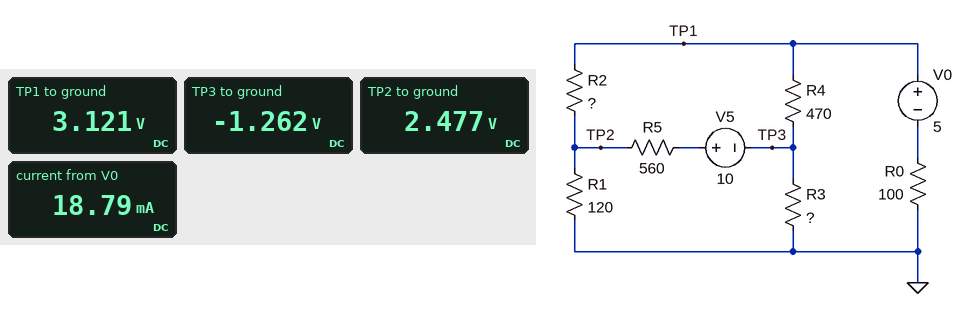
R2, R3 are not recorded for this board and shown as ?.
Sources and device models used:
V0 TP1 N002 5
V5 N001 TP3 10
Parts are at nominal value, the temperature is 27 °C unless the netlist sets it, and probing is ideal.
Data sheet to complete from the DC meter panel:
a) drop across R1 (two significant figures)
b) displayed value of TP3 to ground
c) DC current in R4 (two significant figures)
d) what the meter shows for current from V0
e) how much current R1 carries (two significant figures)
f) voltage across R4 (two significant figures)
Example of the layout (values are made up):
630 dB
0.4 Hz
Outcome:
2.5 V
-1.262 V
9.3 mA
18.79 mA
21 mA
4.4 V
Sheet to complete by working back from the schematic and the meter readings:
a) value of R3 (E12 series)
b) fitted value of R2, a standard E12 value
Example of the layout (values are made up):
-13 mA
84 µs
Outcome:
680 Ω
68 Ω
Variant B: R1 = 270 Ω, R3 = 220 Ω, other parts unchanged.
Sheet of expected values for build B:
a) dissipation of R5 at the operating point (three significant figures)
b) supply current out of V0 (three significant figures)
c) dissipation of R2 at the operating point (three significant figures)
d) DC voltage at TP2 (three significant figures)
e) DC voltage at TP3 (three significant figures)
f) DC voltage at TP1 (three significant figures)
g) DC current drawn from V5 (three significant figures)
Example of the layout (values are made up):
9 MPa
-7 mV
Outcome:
63.9 mW
11.7 mA
528 µW
3.64 V
-381 mV
3.83 V
10.7 mA
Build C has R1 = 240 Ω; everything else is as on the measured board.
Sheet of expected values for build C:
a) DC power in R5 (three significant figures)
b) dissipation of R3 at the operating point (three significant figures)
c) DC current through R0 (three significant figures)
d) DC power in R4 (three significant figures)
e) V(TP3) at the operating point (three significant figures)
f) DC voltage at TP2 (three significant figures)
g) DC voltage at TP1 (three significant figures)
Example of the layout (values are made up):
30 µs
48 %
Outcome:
61.1 mW
777 µW
13.2 mA
41.3 mW
-727 mV
3.42 V
3.68 V
